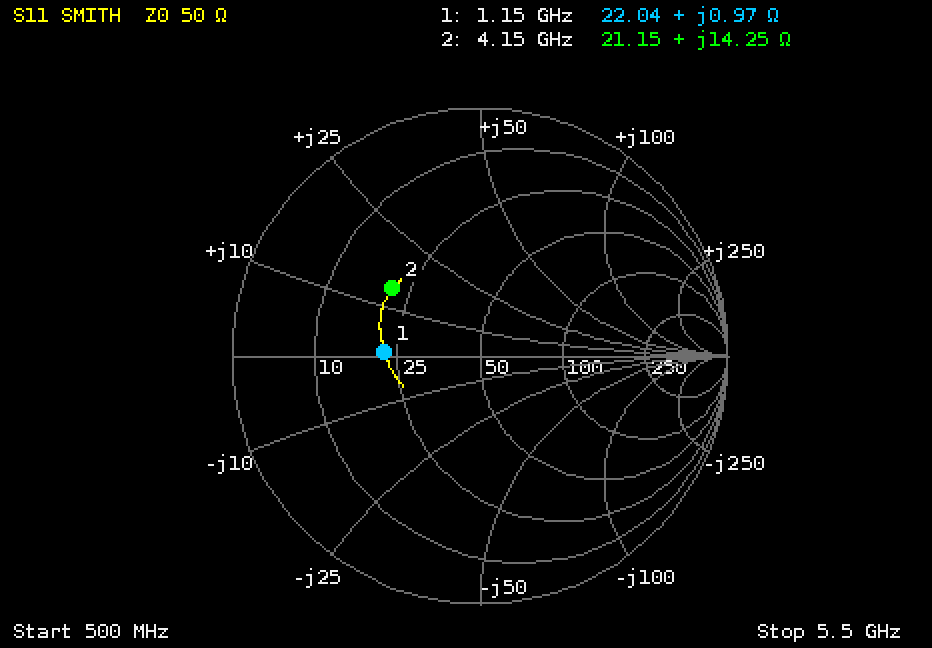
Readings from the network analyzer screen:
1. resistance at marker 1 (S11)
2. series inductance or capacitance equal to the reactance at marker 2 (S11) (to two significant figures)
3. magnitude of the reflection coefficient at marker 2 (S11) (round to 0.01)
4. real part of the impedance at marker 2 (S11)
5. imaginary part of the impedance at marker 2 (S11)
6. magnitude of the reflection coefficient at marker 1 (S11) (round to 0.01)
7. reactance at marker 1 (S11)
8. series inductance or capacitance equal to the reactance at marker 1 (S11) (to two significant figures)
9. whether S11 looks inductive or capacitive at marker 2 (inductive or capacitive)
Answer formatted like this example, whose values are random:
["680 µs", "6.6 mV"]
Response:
["22.04 Ω", "550 pH", "0.44", "21.15 Ω", "+14.25 Ω", "0.39", "+0.97 Ω", "130 pH", "inductive"]
